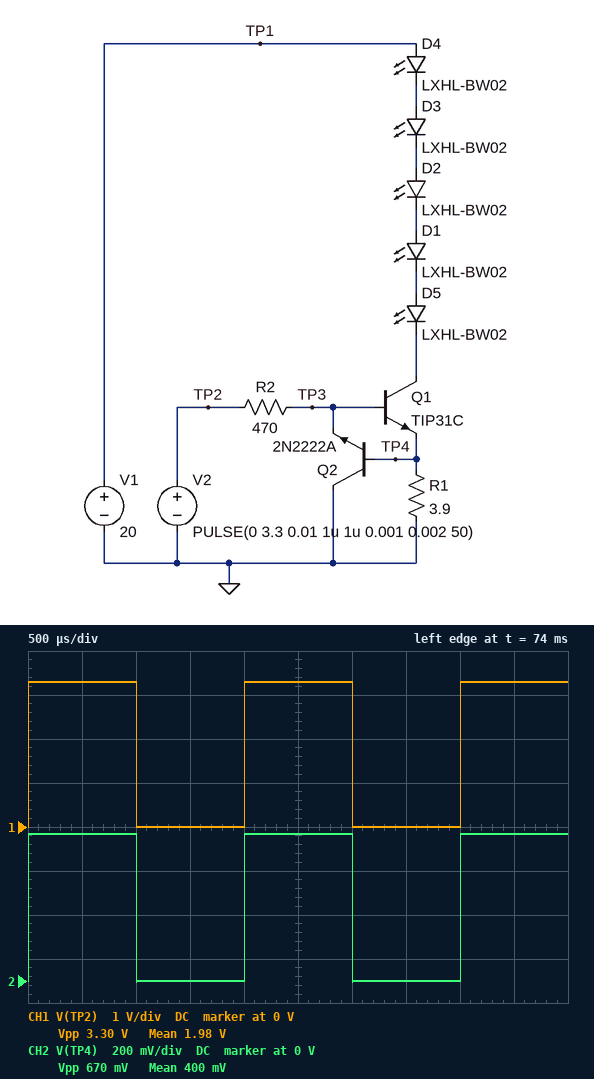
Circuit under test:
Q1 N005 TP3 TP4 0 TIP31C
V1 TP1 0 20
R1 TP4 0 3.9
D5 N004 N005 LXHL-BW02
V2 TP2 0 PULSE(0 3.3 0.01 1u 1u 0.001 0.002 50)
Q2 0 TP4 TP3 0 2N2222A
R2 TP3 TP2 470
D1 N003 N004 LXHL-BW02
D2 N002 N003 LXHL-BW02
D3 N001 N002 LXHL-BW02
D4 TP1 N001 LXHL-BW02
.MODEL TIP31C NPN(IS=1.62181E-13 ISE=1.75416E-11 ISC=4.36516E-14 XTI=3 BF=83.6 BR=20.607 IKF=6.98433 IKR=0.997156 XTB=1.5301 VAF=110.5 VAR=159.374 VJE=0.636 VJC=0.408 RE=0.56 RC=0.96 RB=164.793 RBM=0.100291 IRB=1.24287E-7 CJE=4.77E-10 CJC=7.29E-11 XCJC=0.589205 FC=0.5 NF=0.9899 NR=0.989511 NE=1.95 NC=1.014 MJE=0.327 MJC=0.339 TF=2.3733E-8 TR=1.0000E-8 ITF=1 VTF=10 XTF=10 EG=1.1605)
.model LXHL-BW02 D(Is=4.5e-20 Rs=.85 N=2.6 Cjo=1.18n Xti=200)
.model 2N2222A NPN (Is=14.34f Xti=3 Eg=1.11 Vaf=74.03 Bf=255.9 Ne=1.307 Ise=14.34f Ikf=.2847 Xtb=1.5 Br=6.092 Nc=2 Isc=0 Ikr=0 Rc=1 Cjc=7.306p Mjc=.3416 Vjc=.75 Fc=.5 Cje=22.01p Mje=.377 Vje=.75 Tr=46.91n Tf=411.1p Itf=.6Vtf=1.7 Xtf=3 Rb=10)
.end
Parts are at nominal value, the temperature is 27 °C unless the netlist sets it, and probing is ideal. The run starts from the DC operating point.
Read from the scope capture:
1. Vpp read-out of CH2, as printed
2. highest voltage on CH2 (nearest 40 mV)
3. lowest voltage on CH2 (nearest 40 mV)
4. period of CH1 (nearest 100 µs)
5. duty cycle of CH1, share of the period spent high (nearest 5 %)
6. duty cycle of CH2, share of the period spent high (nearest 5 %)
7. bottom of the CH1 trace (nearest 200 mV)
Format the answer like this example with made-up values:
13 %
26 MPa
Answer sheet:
670 mV
680 mV
0 V
2.0 ms
50 %
50 %
0 V
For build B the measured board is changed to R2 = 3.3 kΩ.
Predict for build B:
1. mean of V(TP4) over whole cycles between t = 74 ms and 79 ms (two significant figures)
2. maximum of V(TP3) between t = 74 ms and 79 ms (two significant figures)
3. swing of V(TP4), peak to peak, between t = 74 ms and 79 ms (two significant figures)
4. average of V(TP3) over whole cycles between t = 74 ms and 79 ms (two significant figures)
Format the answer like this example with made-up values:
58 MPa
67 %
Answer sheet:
120 mV
950 mV
240 mV
480 mV
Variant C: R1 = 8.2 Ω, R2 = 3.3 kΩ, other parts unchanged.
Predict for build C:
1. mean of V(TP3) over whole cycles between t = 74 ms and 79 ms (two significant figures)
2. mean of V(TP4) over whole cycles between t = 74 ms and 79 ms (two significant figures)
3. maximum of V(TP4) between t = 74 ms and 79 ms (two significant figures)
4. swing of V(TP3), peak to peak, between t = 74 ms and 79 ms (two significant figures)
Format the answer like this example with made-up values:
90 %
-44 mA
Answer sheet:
580 mV
230 mV
450 mV
1.2 V
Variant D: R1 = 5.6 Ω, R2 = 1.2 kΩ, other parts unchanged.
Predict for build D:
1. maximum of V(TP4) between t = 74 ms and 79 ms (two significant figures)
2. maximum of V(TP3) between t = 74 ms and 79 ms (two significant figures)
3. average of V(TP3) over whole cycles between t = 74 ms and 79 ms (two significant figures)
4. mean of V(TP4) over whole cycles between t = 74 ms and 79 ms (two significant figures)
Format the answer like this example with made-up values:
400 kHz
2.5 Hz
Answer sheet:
620 mV
1.4 V
690 mV
310 mV
